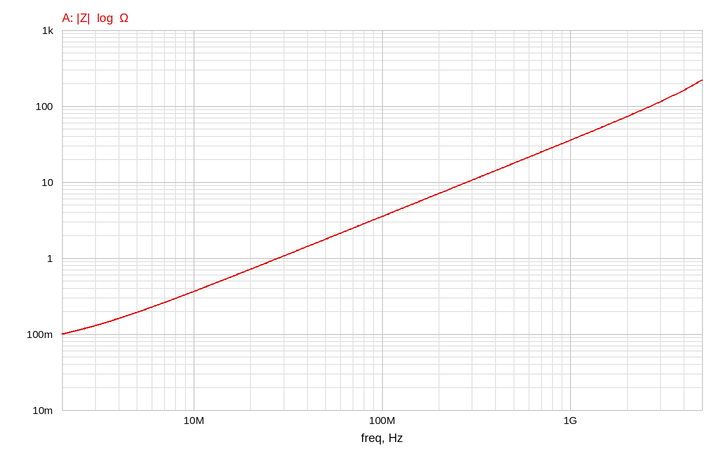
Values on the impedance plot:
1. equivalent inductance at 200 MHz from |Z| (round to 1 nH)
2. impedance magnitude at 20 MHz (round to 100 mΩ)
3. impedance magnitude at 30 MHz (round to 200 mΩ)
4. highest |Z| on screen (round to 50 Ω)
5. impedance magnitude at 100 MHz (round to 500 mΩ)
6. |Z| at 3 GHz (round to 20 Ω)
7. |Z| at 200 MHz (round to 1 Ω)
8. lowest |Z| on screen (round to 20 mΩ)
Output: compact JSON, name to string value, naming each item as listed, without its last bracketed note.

{"equivalent inductance at 200 MHz from |Z|": "6 nH", "impedance magnitude at 20 MHz": "700 mΩ", "impedance magnitude at 30 MHz": "1.0 Ω", "highest |Z| on screen": "200 Ω", "impedance magnitude at 100 MHz": "3.5 Ω", "|Z| at 3 GHz": "120 Ω", "|Z| at 200 MHz": "7 Ω", "lowest |Z| on screen": "100 mΩ"}
